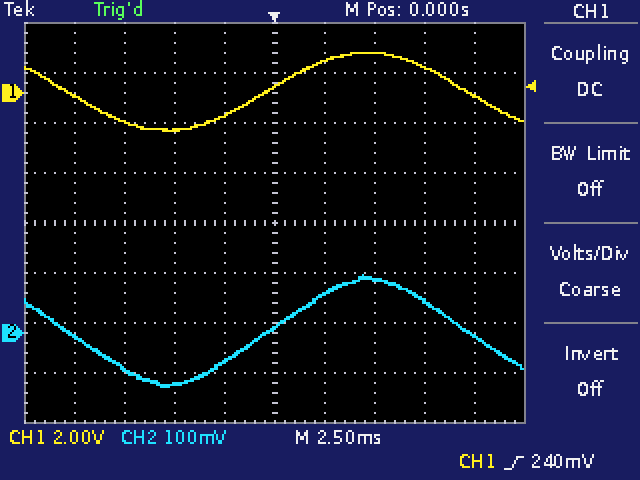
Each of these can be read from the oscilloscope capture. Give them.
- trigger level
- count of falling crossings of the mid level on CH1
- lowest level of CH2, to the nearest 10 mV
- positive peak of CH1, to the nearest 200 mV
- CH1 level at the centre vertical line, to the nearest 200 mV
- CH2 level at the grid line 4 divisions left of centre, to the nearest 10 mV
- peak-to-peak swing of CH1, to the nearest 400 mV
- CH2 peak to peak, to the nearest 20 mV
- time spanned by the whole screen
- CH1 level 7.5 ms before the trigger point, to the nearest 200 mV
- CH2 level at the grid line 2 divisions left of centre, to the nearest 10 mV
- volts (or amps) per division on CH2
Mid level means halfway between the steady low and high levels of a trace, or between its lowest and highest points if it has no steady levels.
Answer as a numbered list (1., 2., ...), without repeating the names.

1. 240 mV
2. 2
3. -110 mV
4. 1.6 V
5. 200 mV
6. -10 mV
7. 3.2 V
8. 220 mV
9. 25 ms
10. -1.2 V
11. -100 mV
12. 100 mV
